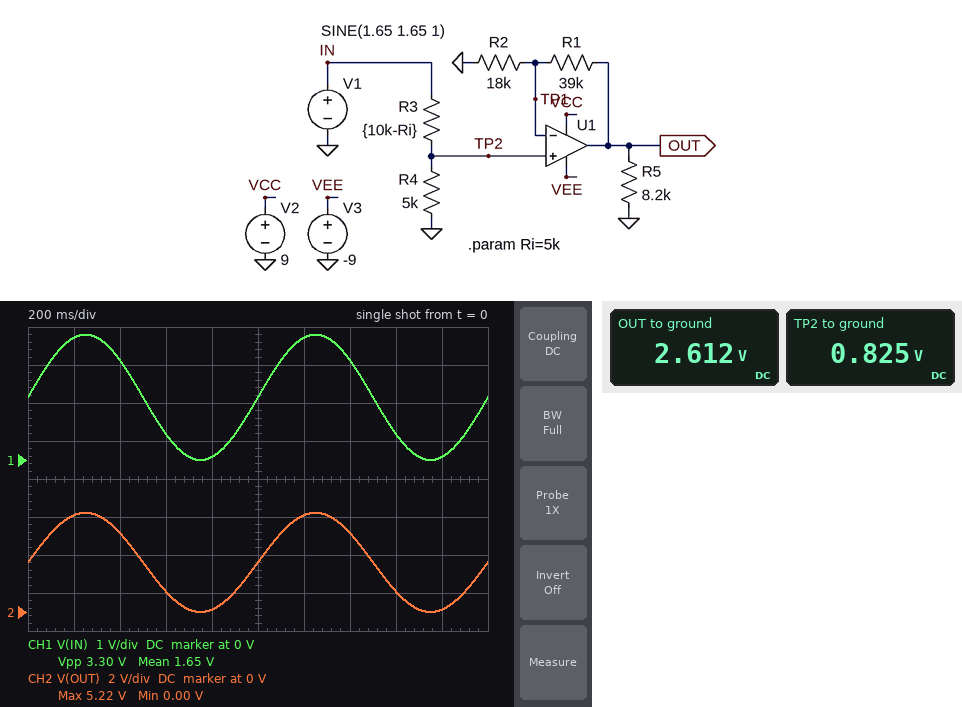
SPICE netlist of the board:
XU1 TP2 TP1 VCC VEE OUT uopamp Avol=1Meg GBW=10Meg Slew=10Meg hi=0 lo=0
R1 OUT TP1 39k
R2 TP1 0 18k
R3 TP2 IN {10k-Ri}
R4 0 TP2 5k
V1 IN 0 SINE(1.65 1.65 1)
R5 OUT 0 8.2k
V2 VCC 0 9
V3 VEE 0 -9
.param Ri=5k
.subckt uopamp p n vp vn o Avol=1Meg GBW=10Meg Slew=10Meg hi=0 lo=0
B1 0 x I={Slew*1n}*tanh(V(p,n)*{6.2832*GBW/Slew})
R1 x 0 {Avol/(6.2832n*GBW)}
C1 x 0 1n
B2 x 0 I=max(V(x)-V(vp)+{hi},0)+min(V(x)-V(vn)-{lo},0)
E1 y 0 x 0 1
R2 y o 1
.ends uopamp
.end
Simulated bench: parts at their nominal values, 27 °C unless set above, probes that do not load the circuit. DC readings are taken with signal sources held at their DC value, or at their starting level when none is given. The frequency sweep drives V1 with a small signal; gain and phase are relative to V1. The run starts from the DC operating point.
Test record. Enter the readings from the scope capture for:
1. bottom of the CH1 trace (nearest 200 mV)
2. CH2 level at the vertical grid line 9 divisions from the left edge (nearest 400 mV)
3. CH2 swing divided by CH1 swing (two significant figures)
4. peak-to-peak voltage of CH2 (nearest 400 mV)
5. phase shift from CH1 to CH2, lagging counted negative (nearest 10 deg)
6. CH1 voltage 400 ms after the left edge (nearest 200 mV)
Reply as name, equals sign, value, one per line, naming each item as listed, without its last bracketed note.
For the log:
bottom of the CH1 trace = 0 V
CH2 level at the vertical grid line 9 divisions from the left edge = 0 V
CH2 swing divided by CH1 swing = 1.6
peak-to-peak voltage of CH2 = 5.2 V
phase shift from CH1 to CH2, lagging counted negative = 0 deg
CH1 voltage 400 ms after the left edge = 2.6 V
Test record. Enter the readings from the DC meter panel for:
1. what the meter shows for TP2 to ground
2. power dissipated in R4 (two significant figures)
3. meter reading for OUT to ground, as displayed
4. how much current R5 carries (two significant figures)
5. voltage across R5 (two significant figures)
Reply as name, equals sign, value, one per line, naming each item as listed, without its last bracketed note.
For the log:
what the meter shows for TP2 to ground = 0.825 V
power dissipated in R4 = 140 µW
meter reading for OUT to ground, as displayed = 2.612 V
how much current R5 carries = 320 µA
voltage across R5 = 2.6 V
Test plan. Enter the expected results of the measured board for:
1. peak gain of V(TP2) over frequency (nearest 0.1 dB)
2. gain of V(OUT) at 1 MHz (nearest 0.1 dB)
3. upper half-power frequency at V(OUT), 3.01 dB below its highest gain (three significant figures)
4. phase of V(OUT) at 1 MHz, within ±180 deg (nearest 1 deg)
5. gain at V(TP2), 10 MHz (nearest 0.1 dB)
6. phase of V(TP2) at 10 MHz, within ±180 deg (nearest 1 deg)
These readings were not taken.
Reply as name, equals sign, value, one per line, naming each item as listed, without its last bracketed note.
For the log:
peak gain of V(TP2) over frequency = -6.0 dB
gain of V(OUT) at 1 MHz = 3.6 dB
upper half-power frequency at V(OUT), 3.01 dB below its highest gain = 3.16 MHz
phase of V(OUT) at 1 MHz, within ±180 deg = -18 deg
gain at V(TP2), 10 MHz = -6.0 dB
phase of V(TP2) at 10 MHz, within ±180 deg = 0 deg
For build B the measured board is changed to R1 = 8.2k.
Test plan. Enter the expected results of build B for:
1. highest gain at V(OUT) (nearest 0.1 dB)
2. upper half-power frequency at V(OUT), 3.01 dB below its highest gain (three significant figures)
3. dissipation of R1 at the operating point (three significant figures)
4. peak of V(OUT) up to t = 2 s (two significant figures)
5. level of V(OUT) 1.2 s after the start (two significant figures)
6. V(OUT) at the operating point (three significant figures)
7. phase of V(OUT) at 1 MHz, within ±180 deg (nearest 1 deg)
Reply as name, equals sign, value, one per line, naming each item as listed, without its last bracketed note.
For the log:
highest gain at V(OUT) = -2.8 dB
upper half-power frequency at V(OUT), 3.01 dB below its highest gain = 6.87 MHz
dissipation of R1 at the operating point = 17.2 µW
peak of V(OUT) up to t = 2 s = 2.4 V
level of V(OUT) 1.2 s after the start = 2.3 V
V(OUT) at the operating point = 1.20 V
phase of V(OUT) at 1 MHz, within ±180 deg = -8 deg
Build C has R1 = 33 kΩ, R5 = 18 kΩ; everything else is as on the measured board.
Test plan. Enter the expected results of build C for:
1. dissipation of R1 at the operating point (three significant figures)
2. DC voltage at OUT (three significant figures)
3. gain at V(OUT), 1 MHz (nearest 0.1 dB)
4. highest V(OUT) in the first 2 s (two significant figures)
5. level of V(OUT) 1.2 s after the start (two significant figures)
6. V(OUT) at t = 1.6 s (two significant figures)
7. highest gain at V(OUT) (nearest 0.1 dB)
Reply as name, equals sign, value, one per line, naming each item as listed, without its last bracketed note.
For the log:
dissipation of R1 at the operating point = 69.3 µW
DC voltage at OUT = 2.34 V
gain at V(OUT), 1 MHz = 2.7 dB
highest V(OUT) in the first 2 s = 4.7 V
level of V(OUT) 1.2 s after the start = 4.6 V
V(OUT) at t = 1.6 s = 960 mV
highest gain at V(OUT) = 3.0 dB
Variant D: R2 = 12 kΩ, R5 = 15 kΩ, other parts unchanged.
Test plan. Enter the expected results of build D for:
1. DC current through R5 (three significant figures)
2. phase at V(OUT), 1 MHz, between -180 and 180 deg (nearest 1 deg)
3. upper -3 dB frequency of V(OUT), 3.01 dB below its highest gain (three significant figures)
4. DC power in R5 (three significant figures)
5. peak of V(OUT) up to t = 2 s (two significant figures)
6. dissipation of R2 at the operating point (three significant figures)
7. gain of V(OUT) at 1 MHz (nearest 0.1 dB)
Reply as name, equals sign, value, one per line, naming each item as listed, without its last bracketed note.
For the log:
DC current through R5 = 234 µA
phase at V(OUT), 1 MHz, between -180 and 180 deg = -23 deg
upper -3 dB frequency of V(OUT), 3.01 dB below its highest gain = 2.35 MHz
DC power in R5 = 820 µW
peak of V(OUT) up to t = 2 s = 7.0 V
dissipation of R2 at the operating point = 56.7 µW
gain of V(OUT) at 1 MHz = 5.8 dB
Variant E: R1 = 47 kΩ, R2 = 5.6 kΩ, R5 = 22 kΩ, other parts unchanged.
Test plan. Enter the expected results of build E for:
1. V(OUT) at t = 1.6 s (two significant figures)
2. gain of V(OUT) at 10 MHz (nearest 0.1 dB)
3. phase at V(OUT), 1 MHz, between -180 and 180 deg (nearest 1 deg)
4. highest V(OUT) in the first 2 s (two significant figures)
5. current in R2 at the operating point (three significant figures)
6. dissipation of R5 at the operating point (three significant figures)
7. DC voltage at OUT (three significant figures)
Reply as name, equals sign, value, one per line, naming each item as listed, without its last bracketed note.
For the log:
V(OUT) at t = 1.6 s = 3.2 V
gain of V(OUT) at 10 MHz = -6.1 dB
phase at V(OUT), 1 MHz, between -180 and 180 deg = -43 deg
highest V(OUT) in the first 2 s = 9.0 V
current in R2 at the operating point = 147 µA
dissipation of R5 at the operating point = 2.73 mW
DC voltage at OUT = 7.75 V
